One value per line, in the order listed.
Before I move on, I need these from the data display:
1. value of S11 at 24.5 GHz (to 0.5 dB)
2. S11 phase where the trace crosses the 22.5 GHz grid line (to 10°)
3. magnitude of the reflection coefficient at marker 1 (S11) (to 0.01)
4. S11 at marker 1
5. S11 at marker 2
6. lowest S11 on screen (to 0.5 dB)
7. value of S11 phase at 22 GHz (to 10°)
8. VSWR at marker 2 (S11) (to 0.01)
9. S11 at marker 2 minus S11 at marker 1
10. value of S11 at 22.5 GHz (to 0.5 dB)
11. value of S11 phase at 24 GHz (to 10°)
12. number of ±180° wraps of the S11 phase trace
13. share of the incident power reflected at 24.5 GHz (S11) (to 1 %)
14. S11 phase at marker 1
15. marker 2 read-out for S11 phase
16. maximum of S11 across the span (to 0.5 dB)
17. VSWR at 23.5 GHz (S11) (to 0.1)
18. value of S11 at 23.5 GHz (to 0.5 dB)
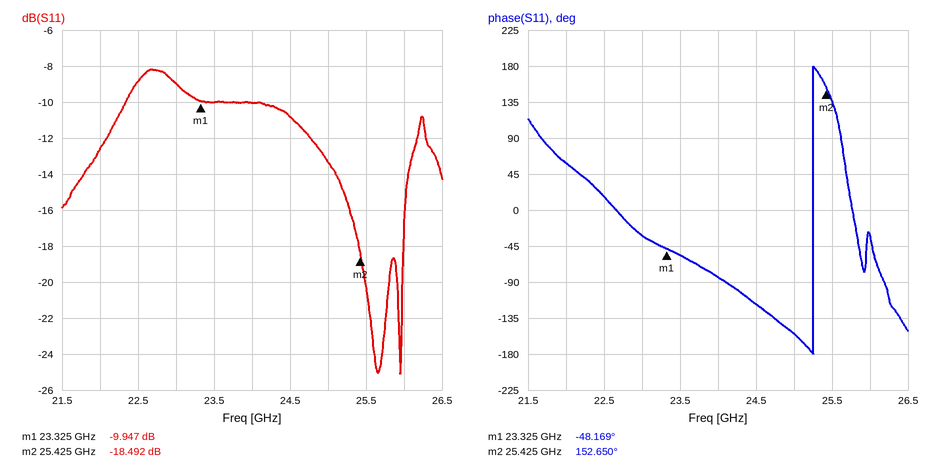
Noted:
-11.0 dB
20°
0.32
-9.947 dB
-18.492 dB
-25.0 dB
60°
1.27
-8.545 dB
-9.0 dB
-80°
1
8 %
-48.169°
152.650°
-8.0 dB
1.9
-10.0 dB
